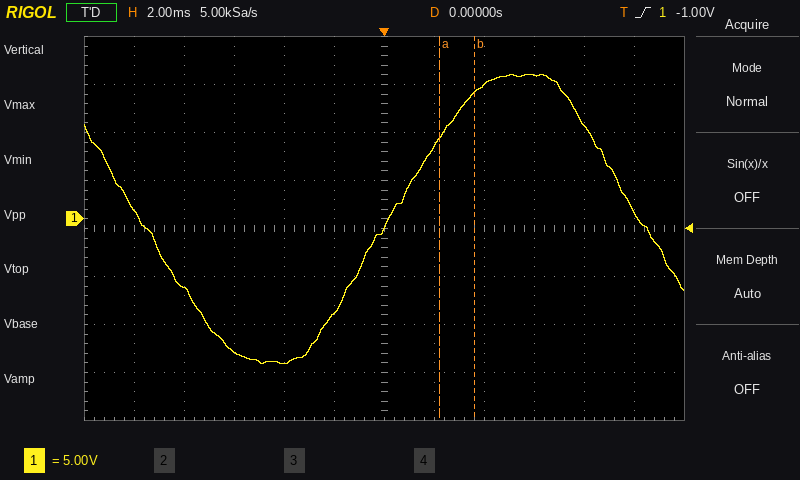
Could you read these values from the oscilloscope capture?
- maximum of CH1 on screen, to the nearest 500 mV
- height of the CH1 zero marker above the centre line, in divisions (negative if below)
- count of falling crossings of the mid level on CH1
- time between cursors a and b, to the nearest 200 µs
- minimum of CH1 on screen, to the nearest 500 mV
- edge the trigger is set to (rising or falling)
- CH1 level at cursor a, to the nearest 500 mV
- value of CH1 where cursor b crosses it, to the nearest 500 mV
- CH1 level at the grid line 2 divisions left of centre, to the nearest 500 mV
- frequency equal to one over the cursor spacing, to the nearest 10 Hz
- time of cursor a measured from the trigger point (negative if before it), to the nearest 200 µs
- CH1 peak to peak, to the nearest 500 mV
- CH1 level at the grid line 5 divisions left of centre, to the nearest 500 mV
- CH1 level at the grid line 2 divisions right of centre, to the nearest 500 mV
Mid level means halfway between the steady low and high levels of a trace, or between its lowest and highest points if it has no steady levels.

15.0 V
+0.2 div
2
1.4 ms
-15.0 V
rising
8.5 V
13.0 V
-15.0 V
710 Hz
+2.2 ms
30.0 V
1.0 V
14.0 V
